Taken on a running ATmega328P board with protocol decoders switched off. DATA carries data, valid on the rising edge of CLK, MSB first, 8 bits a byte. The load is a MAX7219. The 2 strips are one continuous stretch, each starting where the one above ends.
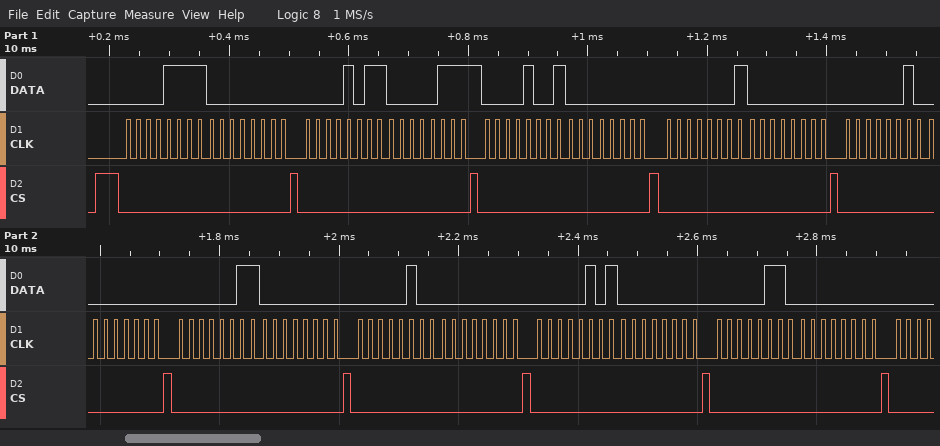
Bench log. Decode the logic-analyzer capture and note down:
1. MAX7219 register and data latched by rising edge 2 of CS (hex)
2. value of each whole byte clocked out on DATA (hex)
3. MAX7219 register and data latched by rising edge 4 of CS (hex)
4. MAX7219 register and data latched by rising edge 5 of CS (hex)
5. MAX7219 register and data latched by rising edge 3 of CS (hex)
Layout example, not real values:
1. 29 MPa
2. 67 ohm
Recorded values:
1. register 0xF, data 0x00
2. 0x0F 0x00 0x0B 0x07 0x09 0x00 0x01 0x00 0x02 0x00 0x03 0x00 0x04 0x00 0x05 0x00 0x06 0x00
3. register 0x9, data 0x00
4. register 0x1, data 0x00
5. register 0xB, data 0x07
